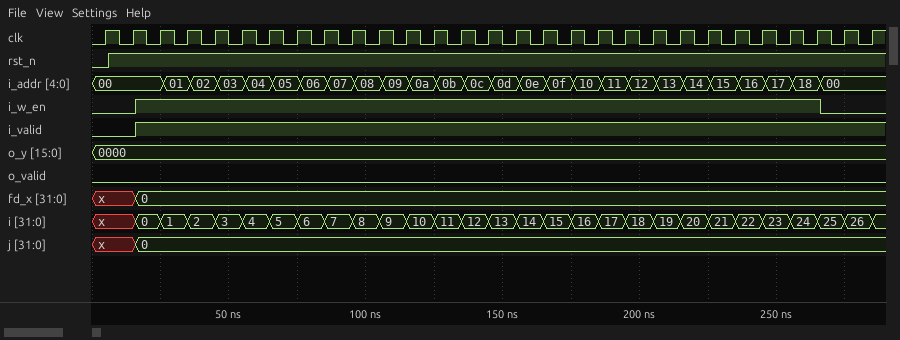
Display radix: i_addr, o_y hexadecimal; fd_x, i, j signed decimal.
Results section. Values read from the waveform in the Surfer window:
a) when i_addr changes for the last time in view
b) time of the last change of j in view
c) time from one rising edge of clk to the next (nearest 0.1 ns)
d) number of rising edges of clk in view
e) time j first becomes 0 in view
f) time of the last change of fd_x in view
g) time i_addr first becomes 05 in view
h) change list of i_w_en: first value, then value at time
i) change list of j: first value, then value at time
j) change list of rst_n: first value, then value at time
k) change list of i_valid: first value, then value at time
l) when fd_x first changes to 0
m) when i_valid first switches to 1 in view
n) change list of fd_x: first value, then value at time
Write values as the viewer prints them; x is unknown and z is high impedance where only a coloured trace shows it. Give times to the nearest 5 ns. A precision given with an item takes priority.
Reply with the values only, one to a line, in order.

265 ns
15 ns
10 ns
29
15 ns
15 ns
65 ns
0, 1 at 15 ns, 0 at 265 ns
x, 0 at 15 ns
0, 1 at 5 ns
0, 1 at 15 ns
15 ns
15 ns
x, 0 at 15 ns
